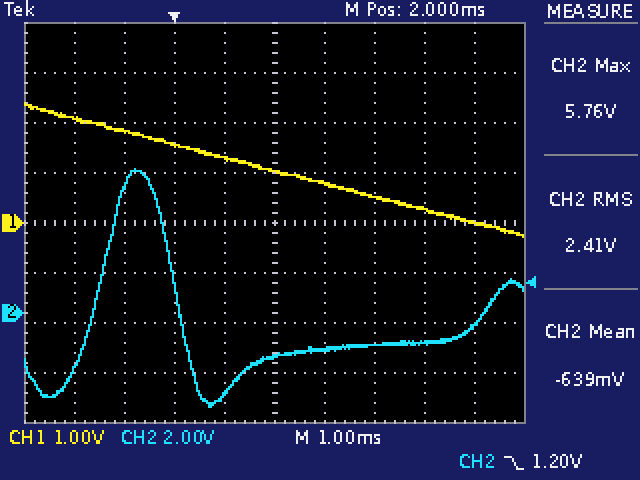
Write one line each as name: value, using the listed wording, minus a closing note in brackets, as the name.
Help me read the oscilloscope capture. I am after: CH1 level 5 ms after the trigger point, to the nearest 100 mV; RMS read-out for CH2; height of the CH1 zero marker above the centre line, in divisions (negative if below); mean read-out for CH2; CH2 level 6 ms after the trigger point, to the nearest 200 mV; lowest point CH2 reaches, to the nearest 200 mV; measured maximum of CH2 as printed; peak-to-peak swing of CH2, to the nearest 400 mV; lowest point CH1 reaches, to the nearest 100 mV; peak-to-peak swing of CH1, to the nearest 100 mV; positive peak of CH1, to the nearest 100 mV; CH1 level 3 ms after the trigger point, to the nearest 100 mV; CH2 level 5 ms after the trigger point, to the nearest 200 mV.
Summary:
CH1 level 5 ms after the trigger point, to the nearest 100 mV: 300 mV
RMS read-out for CH2: 2.41 V
height of the CH1 zero marker above the centre line, in divisions: 0.0 div
mean read-out for CH2: -639 mV
CH2 level 6 ms after the trigger point, to the nearest 200 mV: -400 mV
lowest point CH2 reaches, to the nearest 200 mV: -3.8 V
measured maximum of CH2 as printed: 5.76 V
peak-to-peak swing of CH2, to the nearest 400 mV: 9.6 V
lowest point CH1 reaches, to the nearest 100 mV: -300 mV
peak-to-peak swing of CH1, to the nearest 100 mV: 2.7 V
positive peak of CH1, to the nearest 100 mV: 2.4 V
CH1 level 3 ms after the trigger point, to the nearest 100 mV: 800 mV
CH2 level 5 ms after the trigger point, to the nearest 200 mV: -1.2 V
